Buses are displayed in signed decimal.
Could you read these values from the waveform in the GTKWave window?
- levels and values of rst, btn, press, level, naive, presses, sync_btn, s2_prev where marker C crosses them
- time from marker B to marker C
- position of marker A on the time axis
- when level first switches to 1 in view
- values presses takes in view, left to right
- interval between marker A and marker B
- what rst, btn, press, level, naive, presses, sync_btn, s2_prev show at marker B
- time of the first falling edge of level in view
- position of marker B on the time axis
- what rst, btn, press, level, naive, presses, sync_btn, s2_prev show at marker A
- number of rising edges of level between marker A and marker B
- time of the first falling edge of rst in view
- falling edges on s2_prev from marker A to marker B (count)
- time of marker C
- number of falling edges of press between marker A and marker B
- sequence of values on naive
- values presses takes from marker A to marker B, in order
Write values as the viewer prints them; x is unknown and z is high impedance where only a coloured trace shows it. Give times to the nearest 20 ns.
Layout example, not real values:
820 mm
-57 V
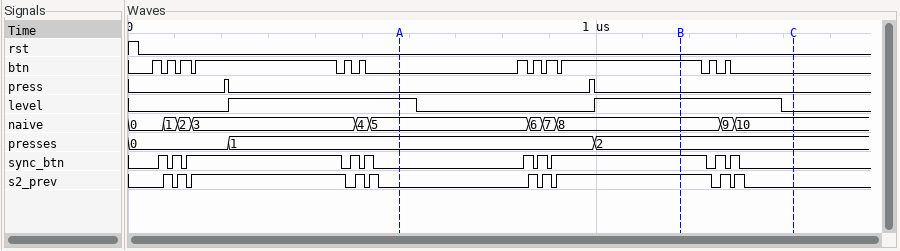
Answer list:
rst=0, btn=0, press=0, level=0, naive=10, presses=2, sync_btn=0, s2_prev=0
240 ns
580 ns
220 ns
0, 1, 2
600 ns
rst=0, btn=1, press=0, level=1, naive=8, presses=2, sync_btn=1, s2_prev=1
620 ns
1180 ns
rst=0, btn=0, press=0, level=1, naive=5, presses=1, sync_btn=0, s2_prev=0
1
20 ns
2
1420 ns
1
0, 1, 2, 3, 4, 5, 6, 7, 8, 9, 10
1, 2
